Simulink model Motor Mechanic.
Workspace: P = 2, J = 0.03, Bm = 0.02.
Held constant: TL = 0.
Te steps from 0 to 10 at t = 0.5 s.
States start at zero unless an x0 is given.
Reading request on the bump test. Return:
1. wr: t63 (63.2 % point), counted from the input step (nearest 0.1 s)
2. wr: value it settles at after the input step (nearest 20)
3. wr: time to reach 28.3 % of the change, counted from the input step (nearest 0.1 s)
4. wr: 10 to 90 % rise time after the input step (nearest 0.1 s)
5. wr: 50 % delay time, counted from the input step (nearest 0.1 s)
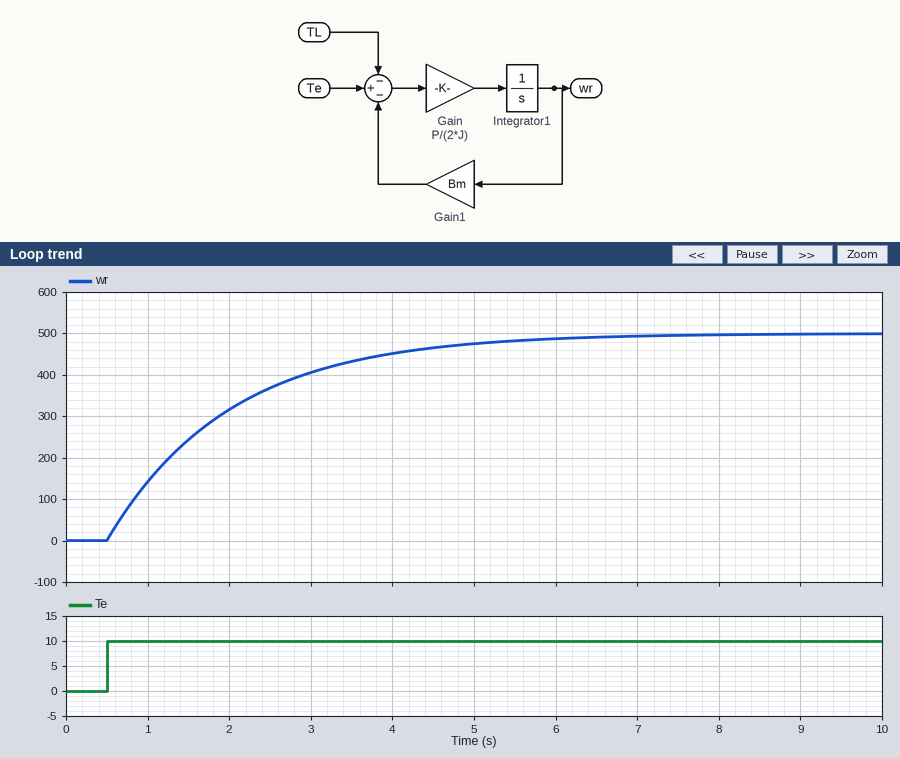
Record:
1.5 s
500
0.5 s
3.3 s
1.0 s
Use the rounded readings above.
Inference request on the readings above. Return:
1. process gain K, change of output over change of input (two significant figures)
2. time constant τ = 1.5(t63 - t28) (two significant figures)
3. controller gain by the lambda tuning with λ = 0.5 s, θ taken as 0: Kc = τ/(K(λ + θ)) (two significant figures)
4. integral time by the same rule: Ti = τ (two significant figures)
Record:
50
1.5 s
0.060
1.5 s
